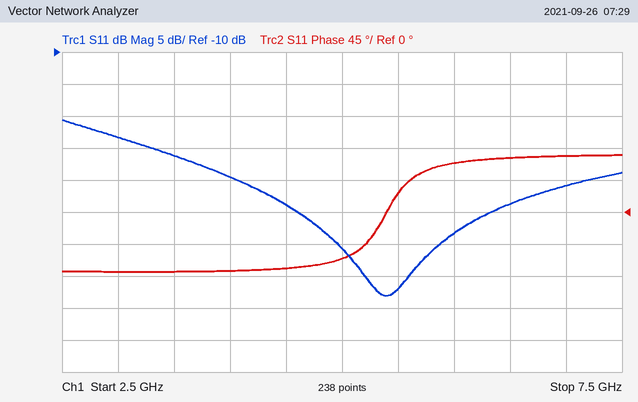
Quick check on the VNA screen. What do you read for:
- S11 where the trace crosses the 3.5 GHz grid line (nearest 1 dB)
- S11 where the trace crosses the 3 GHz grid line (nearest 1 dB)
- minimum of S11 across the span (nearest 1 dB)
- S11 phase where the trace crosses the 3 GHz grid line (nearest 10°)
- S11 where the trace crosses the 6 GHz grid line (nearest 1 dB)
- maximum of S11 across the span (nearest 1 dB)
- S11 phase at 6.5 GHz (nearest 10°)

-26 dB
-23 dB
-48 dB
-80°
-38 dB
-21 dB
80°
